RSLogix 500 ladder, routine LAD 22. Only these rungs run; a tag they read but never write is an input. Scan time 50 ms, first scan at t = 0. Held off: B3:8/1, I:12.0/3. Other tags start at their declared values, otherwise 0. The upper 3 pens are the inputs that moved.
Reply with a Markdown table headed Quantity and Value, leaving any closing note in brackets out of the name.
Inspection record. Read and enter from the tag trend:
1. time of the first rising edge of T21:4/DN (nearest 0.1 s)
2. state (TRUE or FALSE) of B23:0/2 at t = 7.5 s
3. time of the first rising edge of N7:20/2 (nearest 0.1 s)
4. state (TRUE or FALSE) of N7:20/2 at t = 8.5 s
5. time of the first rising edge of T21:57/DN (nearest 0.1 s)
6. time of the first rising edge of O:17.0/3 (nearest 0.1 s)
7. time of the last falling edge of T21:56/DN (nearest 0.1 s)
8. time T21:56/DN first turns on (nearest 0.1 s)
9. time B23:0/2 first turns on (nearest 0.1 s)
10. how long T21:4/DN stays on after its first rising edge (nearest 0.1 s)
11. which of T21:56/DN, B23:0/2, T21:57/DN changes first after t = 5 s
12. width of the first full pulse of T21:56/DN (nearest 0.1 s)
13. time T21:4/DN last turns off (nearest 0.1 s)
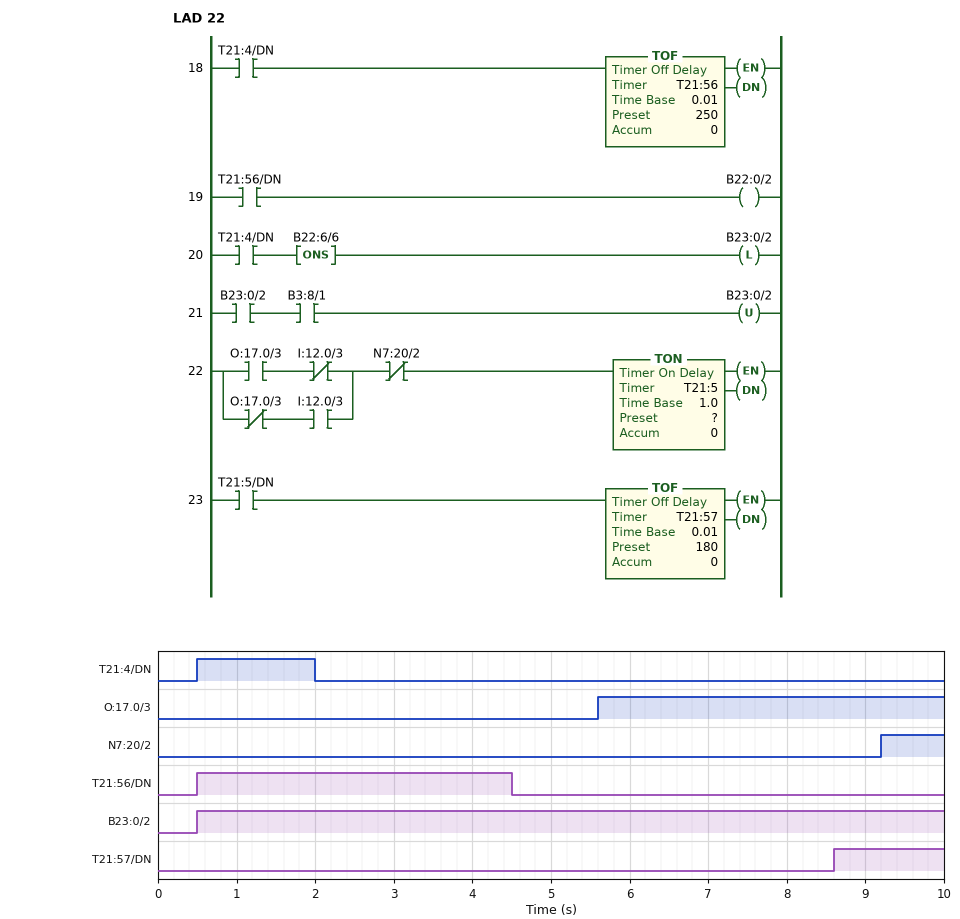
| Quantity | Value |
|---|---|
| time of the first rising edge of T21:4/DN | 0.5 s |
| state (TRUE or FALSE) of B23:0/2 at t = 7.5 s | TRUE |
| time of the first rising edge of N7:20/2 | 9.2 s |
| state (TRUE or FALSE) of N7:20/2 at t = 8.5 s | FALSE |
| time of the first rising edge of T21:57/DN | 8.6 s |
| time of the first rising edge of O:17.0/3 | 5.6 s |
| time of the last falling edge of T21:56/DN | 4.5 s |
| time T21:56/DN first turns on | 0.5 s |
| time B23:0/2 first turns on | 0.5 s |
| how long T21:4/DN stays on after its first rising edge | 1.5 s |
| which of T21:56/DN, B23:0/2, T21:57/DN changes first after t = 5 s | T21:57/DN |
| width of the first full pulse of T21:56/DN | 4.0 s |
| time T21:4/DN last turns off | 2.0 s |
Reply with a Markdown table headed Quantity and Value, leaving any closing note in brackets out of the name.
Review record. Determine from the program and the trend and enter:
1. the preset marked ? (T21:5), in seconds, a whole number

| Quantity | Value |
|---|---|
| the preset marked ? (T21:5), in seconds, a whole number | 3 s |
